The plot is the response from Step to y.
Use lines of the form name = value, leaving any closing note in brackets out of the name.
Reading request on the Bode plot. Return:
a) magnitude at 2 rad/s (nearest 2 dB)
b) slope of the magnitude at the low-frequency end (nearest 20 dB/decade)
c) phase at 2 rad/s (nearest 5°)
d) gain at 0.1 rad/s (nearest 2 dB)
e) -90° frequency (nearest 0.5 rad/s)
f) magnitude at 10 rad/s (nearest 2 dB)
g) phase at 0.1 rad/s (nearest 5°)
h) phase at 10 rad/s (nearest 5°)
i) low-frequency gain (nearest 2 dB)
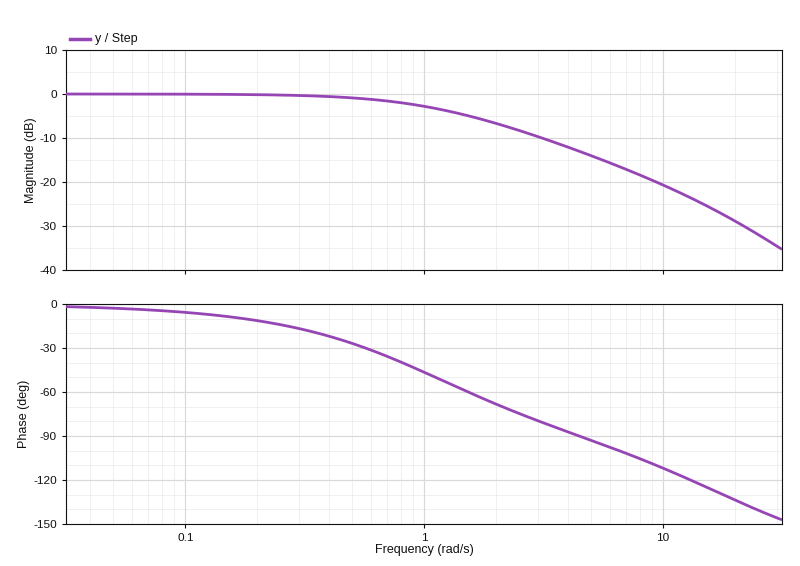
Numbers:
magnitude at 2 rad/s = -6 dB
slope of the magnitude at the low-frequency end = 0 dB/decade
phase at 2 rad/s = -70°
gain at 0.1 rad/s = 0 dB
-90° frequency = 4.5 rad/s
magnitude at 10 rad/s = -20 dB
phase at 0.1 rad/s = -5°
phase at 10 rad/s = -110°
low-frequency gain = 0 dB
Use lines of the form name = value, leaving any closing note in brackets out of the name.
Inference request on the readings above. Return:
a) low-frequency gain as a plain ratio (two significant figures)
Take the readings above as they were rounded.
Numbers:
low-frequency gain as a plain ratio = 1.0
